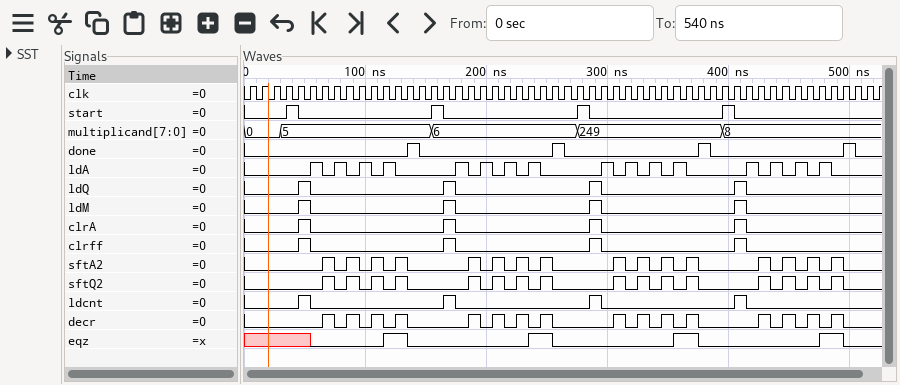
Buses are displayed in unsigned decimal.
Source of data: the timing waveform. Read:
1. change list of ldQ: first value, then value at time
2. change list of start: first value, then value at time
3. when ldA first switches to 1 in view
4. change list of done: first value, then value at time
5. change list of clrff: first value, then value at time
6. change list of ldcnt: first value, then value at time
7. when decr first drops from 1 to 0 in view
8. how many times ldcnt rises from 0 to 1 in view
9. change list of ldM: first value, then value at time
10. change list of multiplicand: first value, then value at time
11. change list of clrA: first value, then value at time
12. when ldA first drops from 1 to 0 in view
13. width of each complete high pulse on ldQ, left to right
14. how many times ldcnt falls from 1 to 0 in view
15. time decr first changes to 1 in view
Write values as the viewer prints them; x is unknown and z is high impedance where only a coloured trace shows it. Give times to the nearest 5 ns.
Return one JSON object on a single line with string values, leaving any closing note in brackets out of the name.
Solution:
{"change list of ldQ: first value, then value at time": "0, 1 at 45 ns, 0 at 55 ns, 1 at 165 ns, 0 at 175 ns, 1 at 285 ns, 0 at 295 ns, 1 at 405 ns, 0 at 415 ns", "change list of start: first value, then value at time": "0, 1 at 35 ns, 0 at 45 ns, 1 at 155 ns, 0 at 165 ns, 1 at 275 ns, 0 at 285 ns, 1 at 395 ns, 0 at 405 ns", "when ldA first switches to 1 in view": "55 ns", "change list of done: first value, then value at time": "0, 1 at 135 ns, 0 at 145 ns, 1 at 255 ns, 0 at 265 ns, 1 at 375 ns, 0 at 385 ns, 1 at 495 ns, 0 at 505 ns", "change list of clrff: first value, then value at time": "0, 1 at 45 ns, 0 at 55 ns, 1 at 165 ns, 0 at 175 ns, 1 at 285 ns, 0 at 295 ns, 1 at 405 ns, 0 at 415 ns", "change list of ldcnt: first value, then value at time": "0, 1 at 45 ns, 0 at 55 ns, 1 at 165 ns, 0 at 175 ns, 1 at 285 ns, 0 at 295 ns, 1 at 405 ns, 0 at 415 ns", "when decr first drops from 1 to 0 in view": "75 ns", "how many times ldcnt rises from 0 to 1 in view": "4", "change list of ldM: first value, then value at time": "0, 1 at 45 ns, 0 at 55 ns, 1 at 165 ns, 0 at 175 ns, 1 at 285 ns, 0 at 295 ns, 1 at 405 ns, 0 at 415 ns", "change list of multiplicand: first value, then value at time": "0, 5 at 30 ns, 6 at 155 ns, 249 at 275 ns, 8 at 395 ns", "change list of clrA: first value, then value at time": "0, 1 at 45 ns, 0 at 55 ns, 1 at 165 ns, 0 at 175 ns, 1 at 285 ns, 0 at 295 ns, 1 at 405 ns, 0 at 415 ns", "when ldA first drops from 1 to 0 in view": "65 ns", "width of each complete high pulse on ldQ, left to right": "10 ns, 10 ns, 10 ns, 10 ns", "how many times ldcnt falls from 1 to 0 in view": "4", "time decr first changes to 1 in view": "65 ns"}
